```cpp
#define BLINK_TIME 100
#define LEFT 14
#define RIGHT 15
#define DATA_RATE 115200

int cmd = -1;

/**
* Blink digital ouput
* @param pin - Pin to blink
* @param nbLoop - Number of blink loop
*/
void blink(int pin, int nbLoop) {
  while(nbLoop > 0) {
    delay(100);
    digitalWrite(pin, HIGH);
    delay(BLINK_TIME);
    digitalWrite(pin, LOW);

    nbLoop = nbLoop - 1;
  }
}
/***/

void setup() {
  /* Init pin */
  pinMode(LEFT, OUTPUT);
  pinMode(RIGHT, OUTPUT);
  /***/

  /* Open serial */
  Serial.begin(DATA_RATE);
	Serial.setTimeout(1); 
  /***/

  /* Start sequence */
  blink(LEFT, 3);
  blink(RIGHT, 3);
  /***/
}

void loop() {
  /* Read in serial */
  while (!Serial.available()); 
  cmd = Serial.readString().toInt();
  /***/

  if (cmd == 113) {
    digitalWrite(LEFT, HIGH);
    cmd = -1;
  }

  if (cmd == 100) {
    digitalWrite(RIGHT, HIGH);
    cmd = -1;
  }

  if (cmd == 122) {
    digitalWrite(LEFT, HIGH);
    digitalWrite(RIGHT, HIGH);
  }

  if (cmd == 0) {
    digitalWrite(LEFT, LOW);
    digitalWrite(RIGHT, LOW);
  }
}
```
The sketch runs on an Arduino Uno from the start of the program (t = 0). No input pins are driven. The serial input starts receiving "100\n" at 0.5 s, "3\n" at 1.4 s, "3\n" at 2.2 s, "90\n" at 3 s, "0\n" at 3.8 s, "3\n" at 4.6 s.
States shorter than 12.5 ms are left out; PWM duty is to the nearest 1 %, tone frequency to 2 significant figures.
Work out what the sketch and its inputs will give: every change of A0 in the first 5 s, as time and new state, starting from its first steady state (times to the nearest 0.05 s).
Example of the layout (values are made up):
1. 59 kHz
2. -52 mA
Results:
1. 0 s low; 0.1 s high; 0.2 s low; 0.3 s high; 0.4 s low; 0.5 s high; 0.6 s low
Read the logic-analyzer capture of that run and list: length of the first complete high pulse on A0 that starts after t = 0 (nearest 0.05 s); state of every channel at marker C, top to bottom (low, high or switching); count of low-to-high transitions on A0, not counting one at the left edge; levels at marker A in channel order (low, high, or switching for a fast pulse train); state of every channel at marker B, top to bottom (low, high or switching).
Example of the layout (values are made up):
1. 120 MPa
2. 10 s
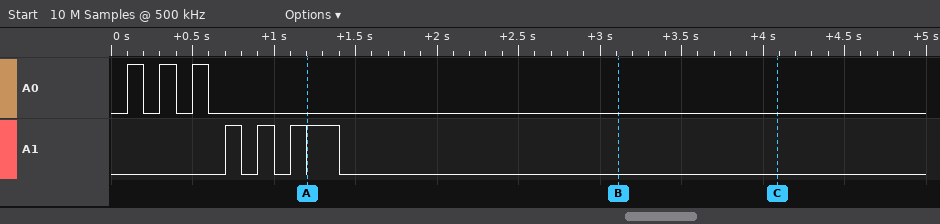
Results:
1. 0.10 s
2. A0 low, A1 low
3. 3
4. A0 low, A1 high
5. A0 low, A1 low
